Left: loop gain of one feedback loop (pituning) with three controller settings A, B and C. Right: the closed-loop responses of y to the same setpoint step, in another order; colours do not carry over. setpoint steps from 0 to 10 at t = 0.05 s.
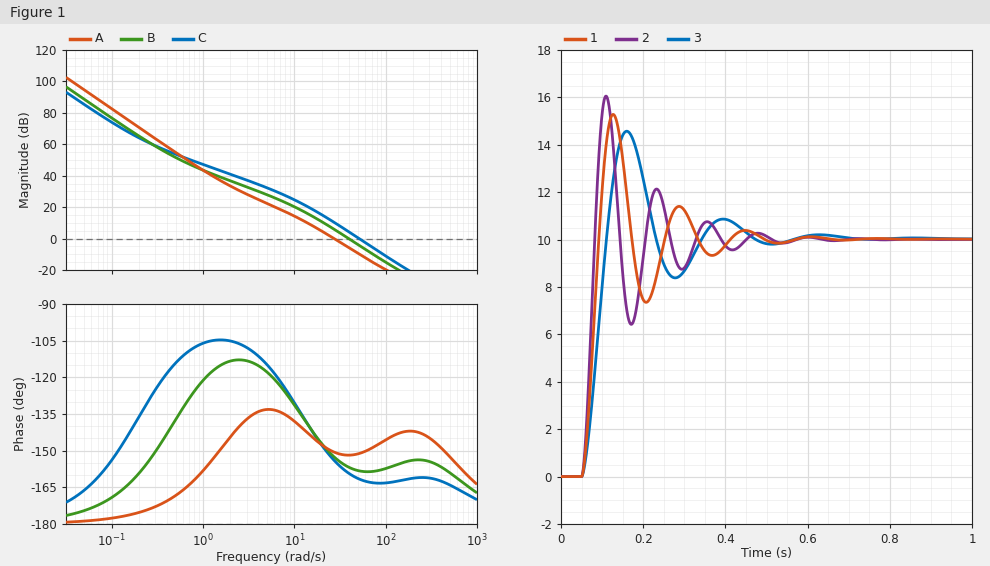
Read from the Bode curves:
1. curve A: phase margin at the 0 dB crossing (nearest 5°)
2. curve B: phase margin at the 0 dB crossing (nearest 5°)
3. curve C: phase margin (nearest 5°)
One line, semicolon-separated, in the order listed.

30°; 25°; 20°
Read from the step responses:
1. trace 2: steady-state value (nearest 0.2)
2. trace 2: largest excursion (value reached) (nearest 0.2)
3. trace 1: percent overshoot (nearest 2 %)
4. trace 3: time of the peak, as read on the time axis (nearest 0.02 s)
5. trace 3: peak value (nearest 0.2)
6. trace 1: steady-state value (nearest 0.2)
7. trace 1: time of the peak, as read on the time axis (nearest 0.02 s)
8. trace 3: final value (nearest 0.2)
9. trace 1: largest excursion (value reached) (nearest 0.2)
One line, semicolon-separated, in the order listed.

10.0; 16.0; 52 %; 0.16 s; 14.6; 10.0; 0.12 s; 10.0; 15.2
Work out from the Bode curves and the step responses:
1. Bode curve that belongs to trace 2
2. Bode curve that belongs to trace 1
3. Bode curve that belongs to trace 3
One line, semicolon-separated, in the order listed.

C; B; A
